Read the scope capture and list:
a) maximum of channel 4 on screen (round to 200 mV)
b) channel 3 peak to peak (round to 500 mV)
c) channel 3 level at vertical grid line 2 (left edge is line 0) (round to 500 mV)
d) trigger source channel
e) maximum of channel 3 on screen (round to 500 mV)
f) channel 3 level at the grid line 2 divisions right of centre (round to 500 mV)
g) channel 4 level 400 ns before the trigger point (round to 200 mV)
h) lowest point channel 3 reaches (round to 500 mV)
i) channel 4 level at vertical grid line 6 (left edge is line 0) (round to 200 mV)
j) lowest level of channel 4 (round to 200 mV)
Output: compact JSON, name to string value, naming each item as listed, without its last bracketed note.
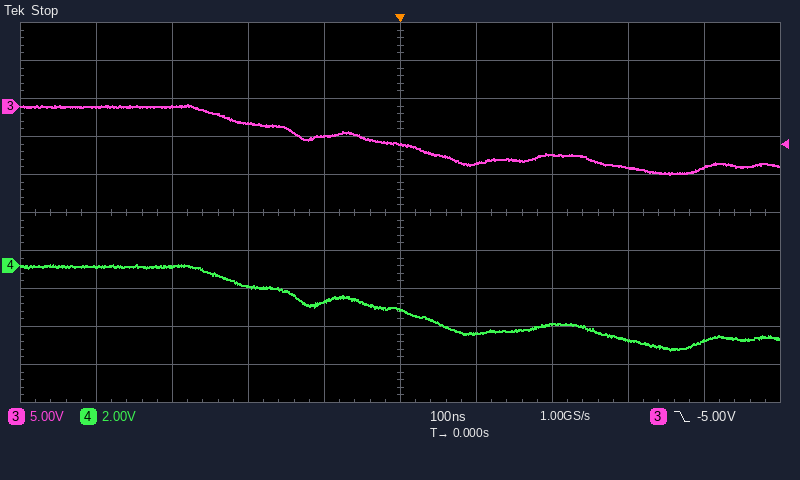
{"maximum of channel 4 on screen": "0.0 V", "channel 3 peak to peak": "9.0 V", "channel 3 level at vertical grid line 2 (left edge is line 0)": "0.0 V", "trigger source channel": "channel 3", "maximum of channel 3 on screen": "0.0 V", "channel 3 level at the grid line 2 divisions right of centre": "-6.5 V", "channel 4 level 400 ns before the trigger point": "0.0 V", "lowest point channel 3 reaches": "-9.0 V", "channel 4 level at vertical grid line 6 (left edge is line 0)": "-3.6 V", "lowest level of channel 4": "-4.4 V"}
